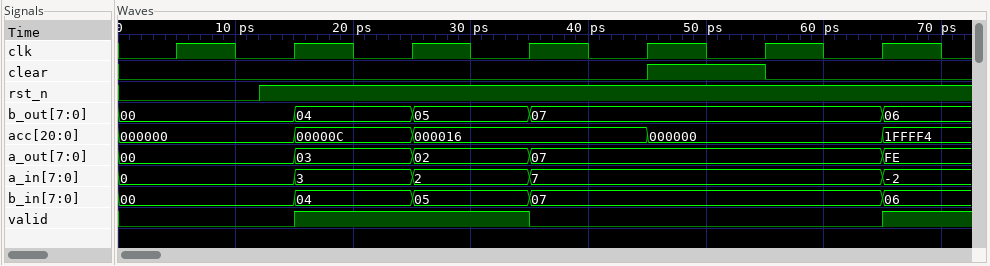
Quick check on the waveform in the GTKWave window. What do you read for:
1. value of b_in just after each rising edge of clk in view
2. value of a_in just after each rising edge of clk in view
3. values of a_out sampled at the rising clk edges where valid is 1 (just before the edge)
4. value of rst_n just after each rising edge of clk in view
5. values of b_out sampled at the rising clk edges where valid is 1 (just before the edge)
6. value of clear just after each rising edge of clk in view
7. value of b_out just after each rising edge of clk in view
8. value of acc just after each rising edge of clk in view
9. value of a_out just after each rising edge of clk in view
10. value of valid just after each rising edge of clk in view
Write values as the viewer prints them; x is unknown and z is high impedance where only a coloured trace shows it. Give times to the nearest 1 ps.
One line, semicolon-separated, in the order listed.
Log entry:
00, 04, 05, 07, 07, 07, 06; 0, 3, 2, 7, 7, 7, -2; 03, 02; 0 1 1 1 1 1 1; 04, 05; 0 0 0 0 1 0 0; 00, 04, 05, 07, 07, 07, 06; 000000, 00000C, 000016, 000016, 000000, 000000, 1FFFF4; 00, 03, 02, 07, 07, 07, FE; 0 1 1 0 0 0 1
